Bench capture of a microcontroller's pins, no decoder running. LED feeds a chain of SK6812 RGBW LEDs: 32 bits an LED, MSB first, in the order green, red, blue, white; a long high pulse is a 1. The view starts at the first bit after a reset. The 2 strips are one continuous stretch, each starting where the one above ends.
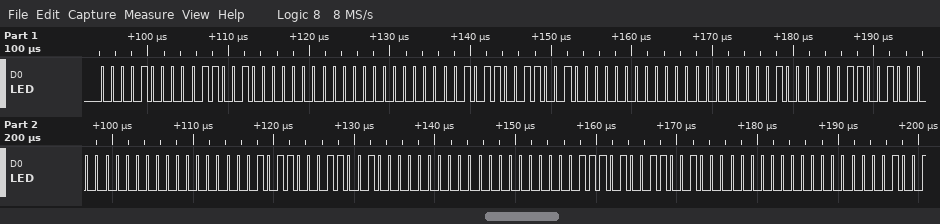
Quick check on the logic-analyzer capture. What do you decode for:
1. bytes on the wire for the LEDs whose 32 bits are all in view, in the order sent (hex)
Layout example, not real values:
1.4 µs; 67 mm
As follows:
08 32 00 00 0B 32 00 00 10 32 00 00 16 32 00 00 1D 32 00 00
